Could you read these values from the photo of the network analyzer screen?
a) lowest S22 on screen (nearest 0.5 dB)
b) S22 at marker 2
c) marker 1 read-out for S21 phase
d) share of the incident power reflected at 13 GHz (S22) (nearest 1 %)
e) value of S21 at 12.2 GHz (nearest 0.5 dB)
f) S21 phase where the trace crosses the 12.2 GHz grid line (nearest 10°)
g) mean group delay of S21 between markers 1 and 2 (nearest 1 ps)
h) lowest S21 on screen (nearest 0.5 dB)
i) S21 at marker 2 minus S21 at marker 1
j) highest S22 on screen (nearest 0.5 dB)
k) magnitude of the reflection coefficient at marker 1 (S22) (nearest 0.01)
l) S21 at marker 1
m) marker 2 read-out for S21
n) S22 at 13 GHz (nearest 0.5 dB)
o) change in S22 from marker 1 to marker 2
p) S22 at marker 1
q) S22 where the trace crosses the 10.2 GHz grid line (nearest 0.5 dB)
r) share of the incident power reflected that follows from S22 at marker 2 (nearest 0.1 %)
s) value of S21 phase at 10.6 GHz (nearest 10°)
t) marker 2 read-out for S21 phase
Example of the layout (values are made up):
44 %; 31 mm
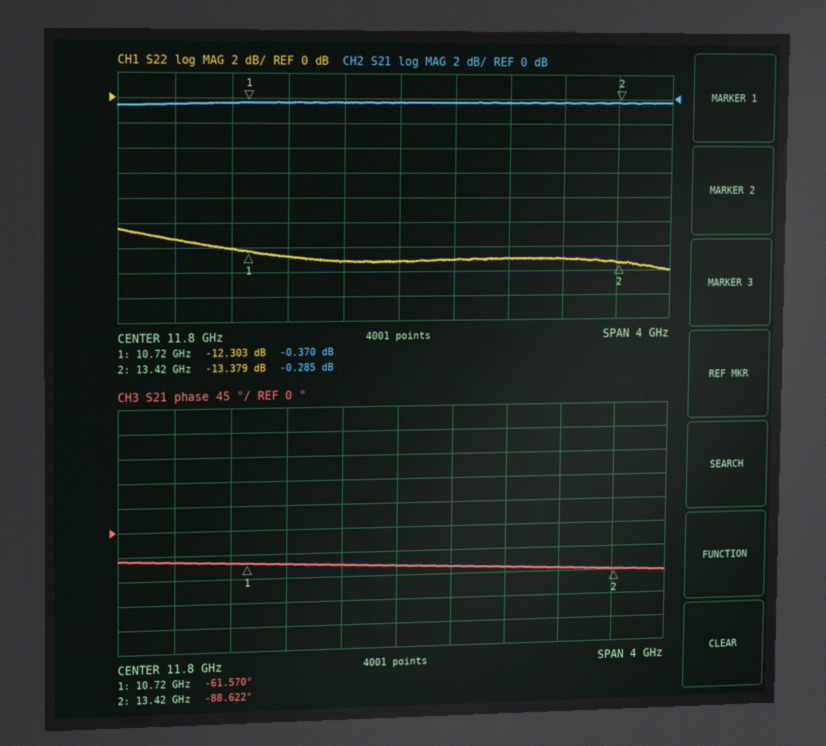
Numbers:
-14.0 dB; -13.379 dB; -61.570°; 5 %; -0.5 dB; -80°; 28 ps; -0.5 dB; 0.085 dB; -10.5 dB; 0.24; -0.370 dB; -0.285 dB; -13.0 dB; -1.076 dB; -12.303 dB; -11.5 dB; 4.6 %; -60°; -88.622°
